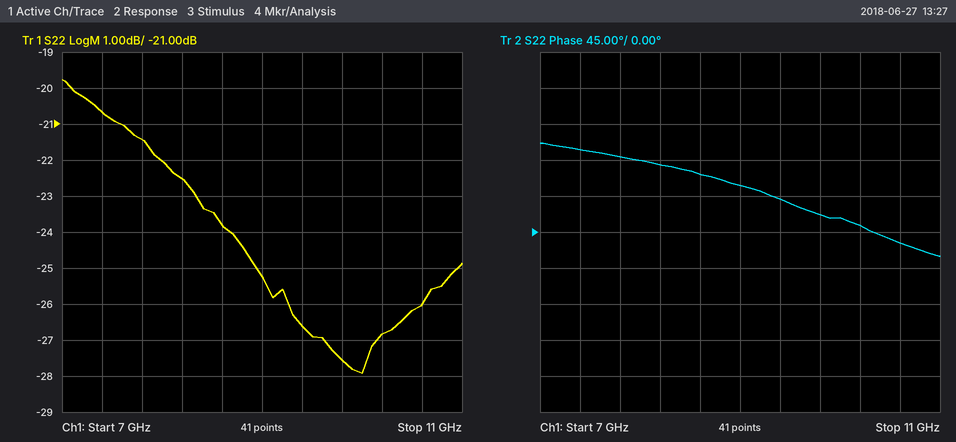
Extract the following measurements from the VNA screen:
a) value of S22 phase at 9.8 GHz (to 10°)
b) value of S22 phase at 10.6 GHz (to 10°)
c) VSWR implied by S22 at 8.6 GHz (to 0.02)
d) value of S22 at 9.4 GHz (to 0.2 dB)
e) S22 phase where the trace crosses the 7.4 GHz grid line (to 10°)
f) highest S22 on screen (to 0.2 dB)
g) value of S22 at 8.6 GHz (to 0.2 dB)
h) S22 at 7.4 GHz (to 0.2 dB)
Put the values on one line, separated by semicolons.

20°; -10°; 1.14; -26.6 dB; 100°; -19.8 dB; -23.8 dB; -20.6 dB
